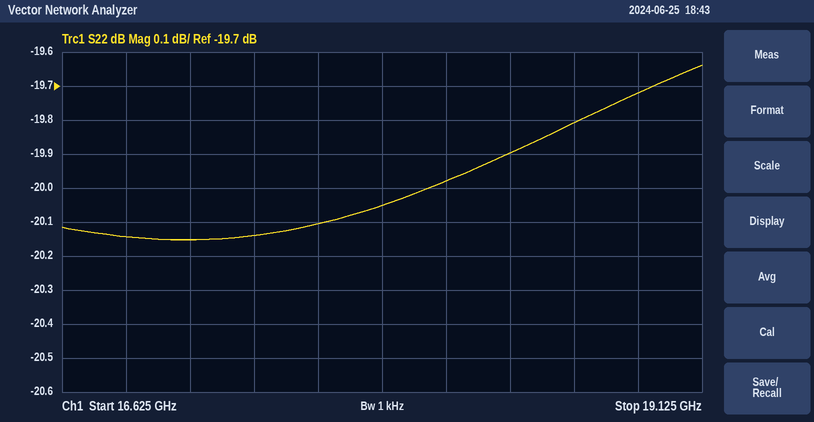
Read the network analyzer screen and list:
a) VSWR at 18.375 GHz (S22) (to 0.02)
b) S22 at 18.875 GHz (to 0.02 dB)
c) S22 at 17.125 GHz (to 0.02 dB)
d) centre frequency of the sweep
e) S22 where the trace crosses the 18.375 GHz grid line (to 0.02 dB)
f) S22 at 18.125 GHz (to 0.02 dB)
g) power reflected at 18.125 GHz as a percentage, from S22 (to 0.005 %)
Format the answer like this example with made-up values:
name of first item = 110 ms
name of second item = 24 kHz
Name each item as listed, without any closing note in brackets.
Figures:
VSWR at 18.375 GHz (S22) = 1.22
S22 at 18.875 GHz = -19.72 dB
S22 at 17.125 GHz = -20.16 dB
centre frequency of the sweep = 17.875 GHz
S22 where the trace crosses the 18.375 GHz grid line = -19.90 dB
S22 at 18.125 GHz = -19.98 dB
power reflected at 18.125 GHz as a percentage, from S22 = 1.005 %
